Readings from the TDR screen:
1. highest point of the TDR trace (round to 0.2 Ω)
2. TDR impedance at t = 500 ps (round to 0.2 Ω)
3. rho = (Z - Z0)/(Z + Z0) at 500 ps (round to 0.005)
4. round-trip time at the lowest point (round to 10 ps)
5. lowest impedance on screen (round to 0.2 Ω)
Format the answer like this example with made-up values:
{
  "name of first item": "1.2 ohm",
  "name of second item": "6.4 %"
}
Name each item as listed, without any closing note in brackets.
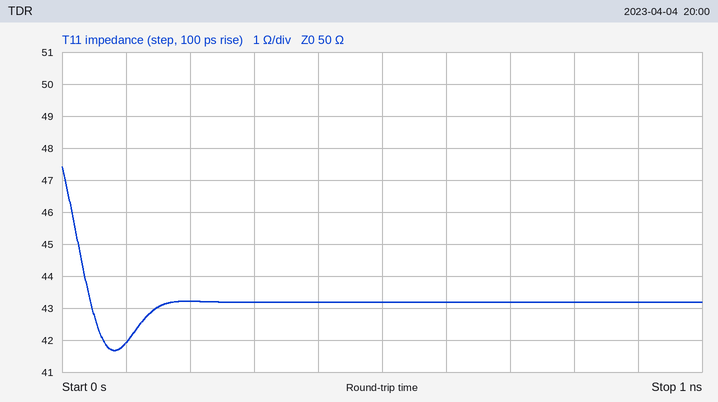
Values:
{
  "highest point of the TDR trace": "47.4 Ω",
  "TDR impedance at t = 500 ps": "43.2 Ω",
  "rho = (Z - Z0)/(Z + Z0) at 500 ps": "-0.075",
  "round-trip time at the lowest point": "80 ps",
  "lowest impedance on screen": "41.6 Ω"
}
